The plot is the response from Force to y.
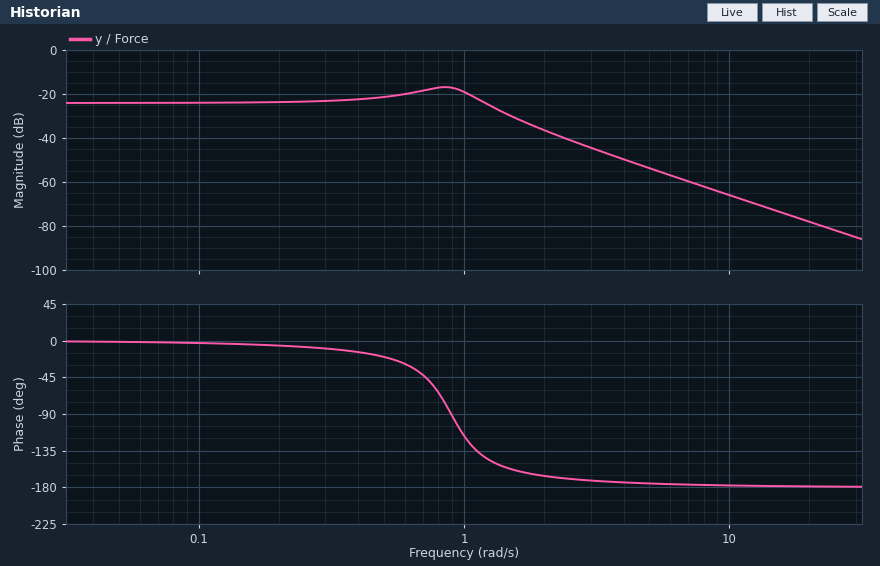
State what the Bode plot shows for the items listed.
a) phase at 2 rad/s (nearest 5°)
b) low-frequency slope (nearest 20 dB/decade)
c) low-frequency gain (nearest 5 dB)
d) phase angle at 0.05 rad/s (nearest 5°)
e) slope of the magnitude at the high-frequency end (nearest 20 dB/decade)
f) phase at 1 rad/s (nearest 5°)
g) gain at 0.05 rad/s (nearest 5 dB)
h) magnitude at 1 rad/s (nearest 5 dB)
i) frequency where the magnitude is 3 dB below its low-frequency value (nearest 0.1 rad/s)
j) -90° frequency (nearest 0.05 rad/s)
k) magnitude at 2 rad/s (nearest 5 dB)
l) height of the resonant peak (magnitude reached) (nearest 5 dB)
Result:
-165°
0 dB/decade
-25 dB
0°
-40 dB/decade
-115°
-25 dB
-20 dB
1.3 rad/s
0.90 rad/s
-35 dB
-15 dB
